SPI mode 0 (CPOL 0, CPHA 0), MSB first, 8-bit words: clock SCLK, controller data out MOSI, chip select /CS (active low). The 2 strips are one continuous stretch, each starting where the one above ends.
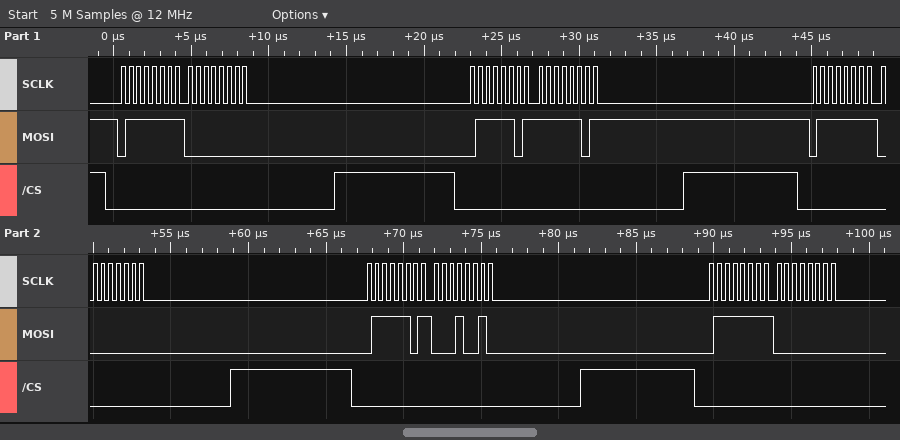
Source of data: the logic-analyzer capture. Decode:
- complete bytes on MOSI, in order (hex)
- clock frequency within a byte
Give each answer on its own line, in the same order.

7F 00 7D FD 7F 00 7D 12 7F 00
2 MHz
